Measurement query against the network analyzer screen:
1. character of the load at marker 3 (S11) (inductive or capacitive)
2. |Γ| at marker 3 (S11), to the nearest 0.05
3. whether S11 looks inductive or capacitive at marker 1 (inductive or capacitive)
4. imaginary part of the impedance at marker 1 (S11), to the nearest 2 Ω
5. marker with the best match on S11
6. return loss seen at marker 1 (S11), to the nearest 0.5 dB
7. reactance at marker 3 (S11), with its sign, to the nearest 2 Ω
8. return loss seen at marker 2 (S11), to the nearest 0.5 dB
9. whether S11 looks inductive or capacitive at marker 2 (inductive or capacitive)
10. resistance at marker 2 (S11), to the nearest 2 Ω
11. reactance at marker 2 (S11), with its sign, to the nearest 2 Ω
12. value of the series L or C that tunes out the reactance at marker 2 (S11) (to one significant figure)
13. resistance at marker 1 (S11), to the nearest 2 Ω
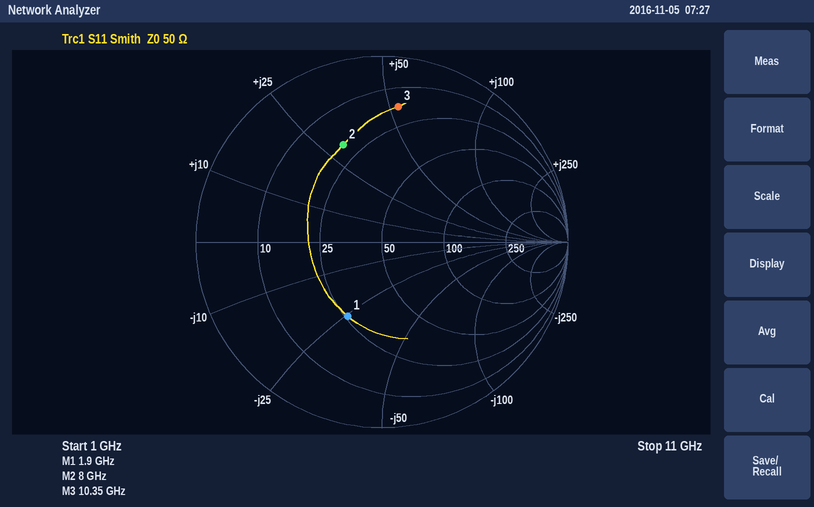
inductive
0.75
capacitive
-26 Ω
marker 1
7.0 dB
+54 Ω
5.0 dB
inductive
20 Ω
+30 Ω
700 fF
26 Ω
